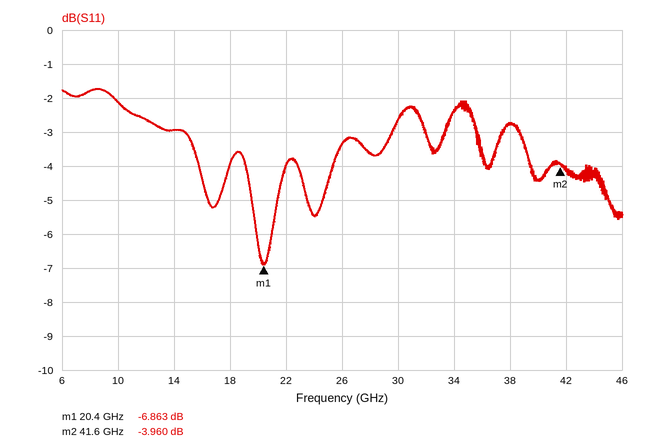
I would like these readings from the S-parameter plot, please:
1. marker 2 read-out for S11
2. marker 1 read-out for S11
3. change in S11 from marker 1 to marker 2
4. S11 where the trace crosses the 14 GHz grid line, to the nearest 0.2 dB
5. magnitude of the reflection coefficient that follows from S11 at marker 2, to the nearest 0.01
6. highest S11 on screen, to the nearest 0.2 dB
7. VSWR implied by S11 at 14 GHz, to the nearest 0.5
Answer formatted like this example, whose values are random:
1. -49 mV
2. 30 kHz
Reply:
1. -3.960 dB
2. -6.863 dB
3. 2.903 dB
4. -3.0 dB
5. 0.63
6. -1.8 dB
7. 6.0
